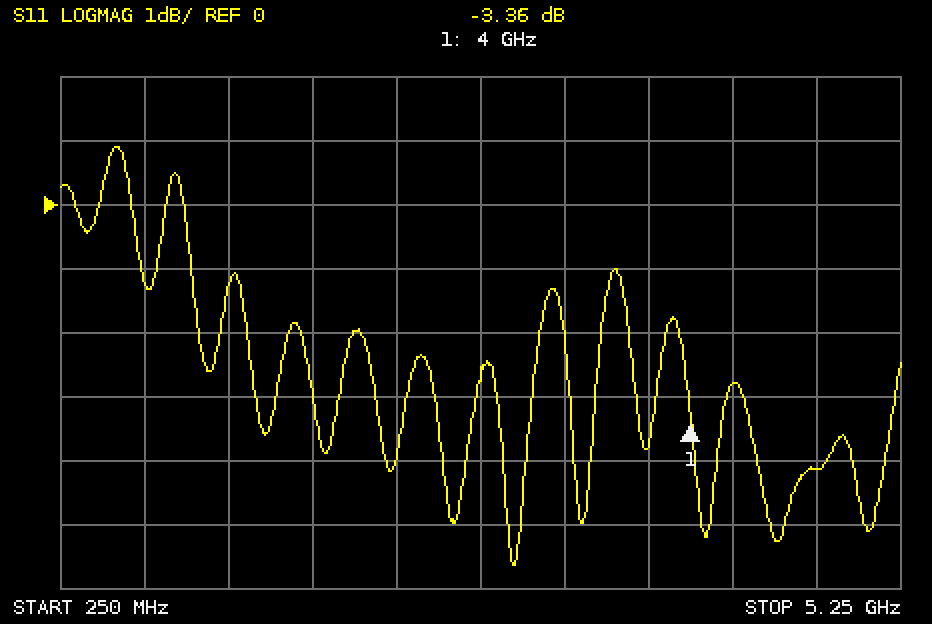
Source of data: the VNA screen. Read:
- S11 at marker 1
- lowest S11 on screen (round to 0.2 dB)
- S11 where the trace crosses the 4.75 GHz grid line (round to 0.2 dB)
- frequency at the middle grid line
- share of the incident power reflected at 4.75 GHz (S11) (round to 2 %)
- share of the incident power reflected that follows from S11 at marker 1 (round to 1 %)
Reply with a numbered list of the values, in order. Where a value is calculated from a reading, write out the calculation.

1. -3.36 dB
2. -5.6 dB
3. -4.2 dB
4. 2.75 GHz
5. 10^(-4.2/10) ≈ 38 %
6. 10^(-3.36/10) ≈ 46 %
